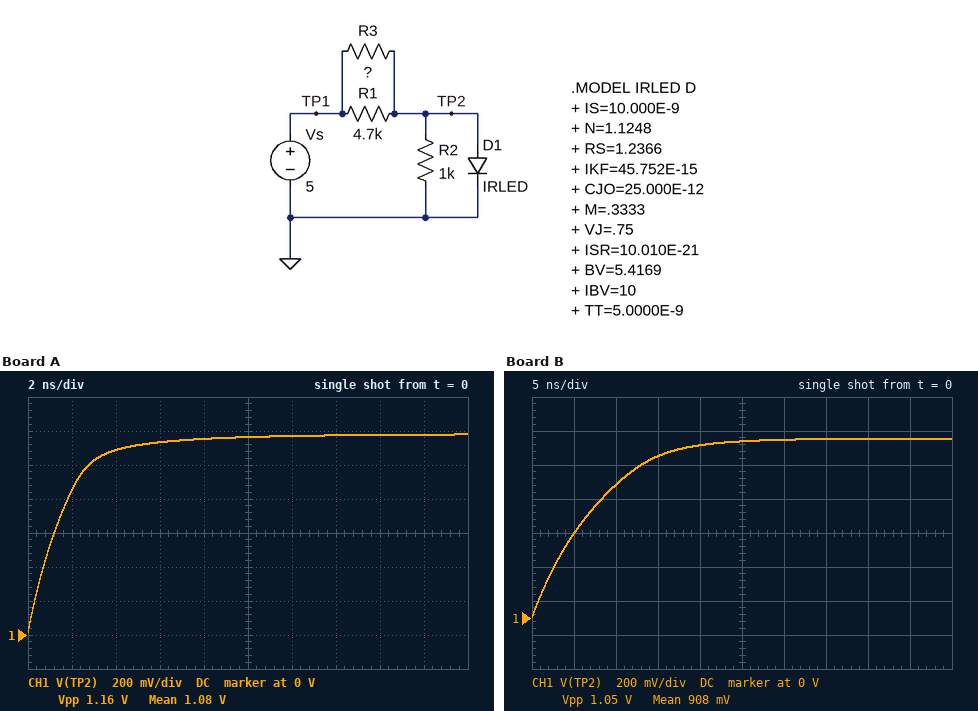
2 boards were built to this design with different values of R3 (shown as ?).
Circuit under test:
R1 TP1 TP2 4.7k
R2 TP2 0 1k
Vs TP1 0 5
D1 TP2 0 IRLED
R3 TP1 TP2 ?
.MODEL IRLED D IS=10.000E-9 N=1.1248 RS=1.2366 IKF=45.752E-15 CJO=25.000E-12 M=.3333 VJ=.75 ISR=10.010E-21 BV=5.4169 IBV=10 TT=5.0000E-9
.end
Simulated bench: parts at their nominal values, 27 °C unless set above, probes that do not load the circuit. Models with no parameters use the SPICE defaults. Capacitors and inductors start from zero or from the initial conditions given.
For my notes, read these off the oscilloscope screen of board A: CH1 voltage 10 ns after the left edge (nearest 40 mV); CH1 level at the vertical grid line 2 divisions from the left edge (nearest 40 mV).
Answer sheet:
1.16 V
1.08 V
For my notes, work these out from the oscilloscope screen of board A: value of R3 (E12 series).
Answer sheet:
330 Ω
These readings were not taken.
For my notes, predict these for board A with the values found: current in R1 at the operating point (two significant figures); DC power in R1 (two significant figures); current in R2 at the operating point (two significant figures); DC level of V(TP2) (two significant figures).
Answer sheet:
810 µA
3.1 mW
1.2 mA
1.2 V
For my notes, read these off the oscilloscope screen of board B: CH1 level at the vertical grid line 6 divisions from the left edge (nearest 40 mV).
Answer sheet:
1.04 V
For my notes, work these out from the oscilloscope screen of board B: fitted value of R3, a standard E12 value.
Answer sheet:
2.2 kΩ
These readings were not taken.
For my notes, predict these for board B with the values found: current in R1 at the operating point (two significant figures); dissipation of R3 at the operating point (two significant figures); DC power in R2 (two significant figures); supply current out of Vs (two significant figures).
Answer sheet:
840 µA
7.1 mW
1.1 mW
2.6 mA
